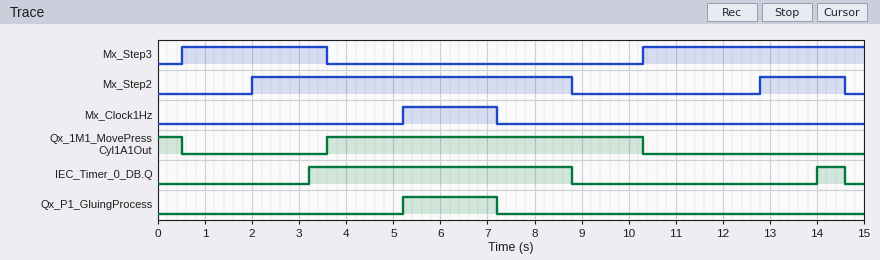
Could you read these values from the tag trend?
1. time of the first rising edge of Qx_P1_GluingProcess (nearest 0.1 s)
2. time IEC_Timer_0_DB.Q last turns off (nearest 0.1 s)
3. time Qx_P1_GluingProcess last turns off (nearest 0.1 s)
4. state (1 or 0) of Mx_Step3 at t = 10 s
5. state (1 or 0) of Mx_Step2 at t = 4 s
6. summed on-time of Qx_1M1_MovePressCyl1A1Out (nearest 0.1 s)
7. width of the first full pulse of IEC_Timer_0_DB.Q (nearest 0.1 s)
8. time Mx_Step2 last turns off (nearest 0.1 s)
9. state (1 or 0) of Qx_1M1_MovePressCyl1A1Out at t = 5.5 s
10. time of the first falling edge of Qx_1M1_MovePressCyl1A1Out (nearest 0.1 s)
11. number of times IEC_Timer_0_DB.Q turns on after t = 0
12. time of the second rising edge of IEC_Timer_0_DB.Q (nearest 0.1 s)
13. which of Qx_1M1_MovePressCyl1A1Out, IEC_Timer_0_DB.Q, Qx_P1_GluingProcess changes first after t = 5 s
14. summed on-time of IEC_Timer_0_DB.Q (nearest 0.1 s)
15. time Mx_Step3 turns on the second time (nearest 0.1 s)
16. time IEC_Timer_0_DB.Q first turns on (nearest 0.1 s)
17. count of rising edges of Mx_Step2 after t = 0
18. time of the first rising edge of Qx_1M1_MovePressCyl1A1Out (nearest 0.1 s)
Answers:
5.2 s
14.6 s
7.2 s
0
1
7.2 s
5.6 s
14.6 s
1
0.5 s
2
14.0 s
Qx_P1_GluingProcess
6.2 s
10.3 s
3.2 s
2
3.6 s
